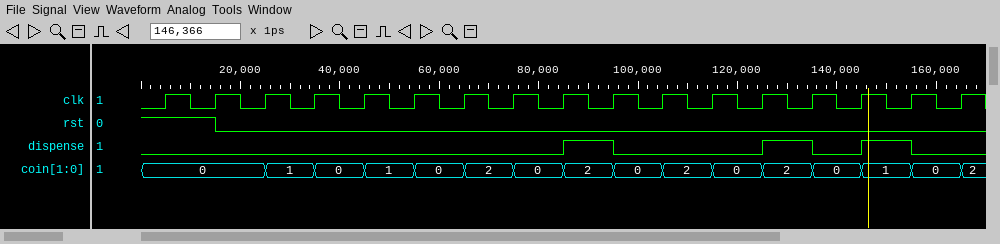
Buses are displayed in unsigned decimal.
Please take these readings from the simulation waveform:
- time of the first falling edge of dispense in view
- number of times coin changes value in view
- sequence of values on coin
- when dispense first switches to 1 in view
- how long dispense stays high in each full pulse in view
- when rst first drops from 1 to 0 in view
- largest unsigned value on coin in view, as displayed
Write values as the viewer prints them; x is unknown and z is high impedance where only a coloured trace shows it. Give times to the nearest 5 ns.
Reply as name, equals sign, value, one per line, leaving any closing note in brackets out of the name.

time of the first falling edge of dispense in view = 95 ns
number of times coin changes value in view = 15
sequence of values on coin = 0, 1, 0, 1, 0, 2, 0, 2, 0, 2, 0, 2, 0, 1, 0, 2
when dispense first switches to 1 in view = 85 ns
how long dispense stays high in each full pulse in view = 10 ns, 10 ns, 10 ns
when rst first drops from 1 to 0 in view = 15 ns
largest unsigned value on coin in view, as displayed = 2
